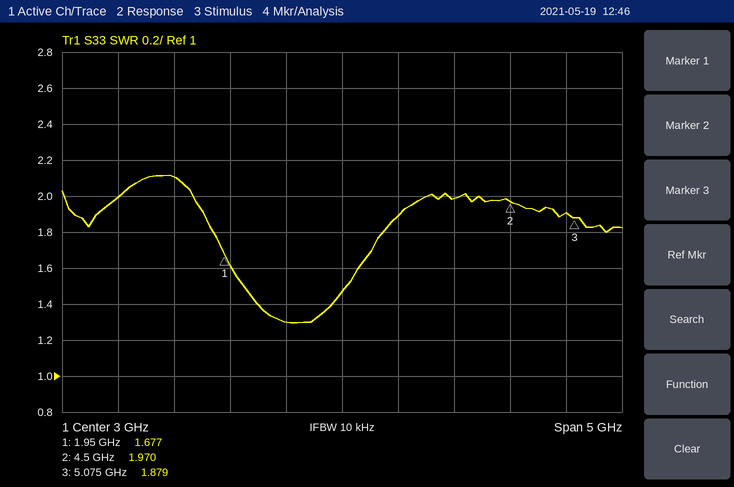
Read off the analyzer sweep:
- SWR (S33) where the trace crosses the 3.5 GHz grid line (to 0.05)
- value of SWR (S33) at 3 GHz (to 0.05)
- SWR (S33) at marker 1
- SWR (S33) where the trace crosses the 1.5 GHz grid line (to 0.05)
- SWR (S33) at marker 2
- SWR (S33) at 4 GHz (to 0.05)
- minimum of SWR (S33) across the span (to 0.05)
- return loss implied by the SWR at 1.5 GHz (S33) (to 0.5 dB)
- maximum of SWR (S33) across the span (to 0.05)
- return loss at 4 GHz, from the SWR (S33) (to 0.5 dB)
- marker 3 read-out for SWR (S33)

1.90
1.45
1.677
2.10
1.970
2.00
1.30
9.0 dB
2.10
9.5 dB
1.879
